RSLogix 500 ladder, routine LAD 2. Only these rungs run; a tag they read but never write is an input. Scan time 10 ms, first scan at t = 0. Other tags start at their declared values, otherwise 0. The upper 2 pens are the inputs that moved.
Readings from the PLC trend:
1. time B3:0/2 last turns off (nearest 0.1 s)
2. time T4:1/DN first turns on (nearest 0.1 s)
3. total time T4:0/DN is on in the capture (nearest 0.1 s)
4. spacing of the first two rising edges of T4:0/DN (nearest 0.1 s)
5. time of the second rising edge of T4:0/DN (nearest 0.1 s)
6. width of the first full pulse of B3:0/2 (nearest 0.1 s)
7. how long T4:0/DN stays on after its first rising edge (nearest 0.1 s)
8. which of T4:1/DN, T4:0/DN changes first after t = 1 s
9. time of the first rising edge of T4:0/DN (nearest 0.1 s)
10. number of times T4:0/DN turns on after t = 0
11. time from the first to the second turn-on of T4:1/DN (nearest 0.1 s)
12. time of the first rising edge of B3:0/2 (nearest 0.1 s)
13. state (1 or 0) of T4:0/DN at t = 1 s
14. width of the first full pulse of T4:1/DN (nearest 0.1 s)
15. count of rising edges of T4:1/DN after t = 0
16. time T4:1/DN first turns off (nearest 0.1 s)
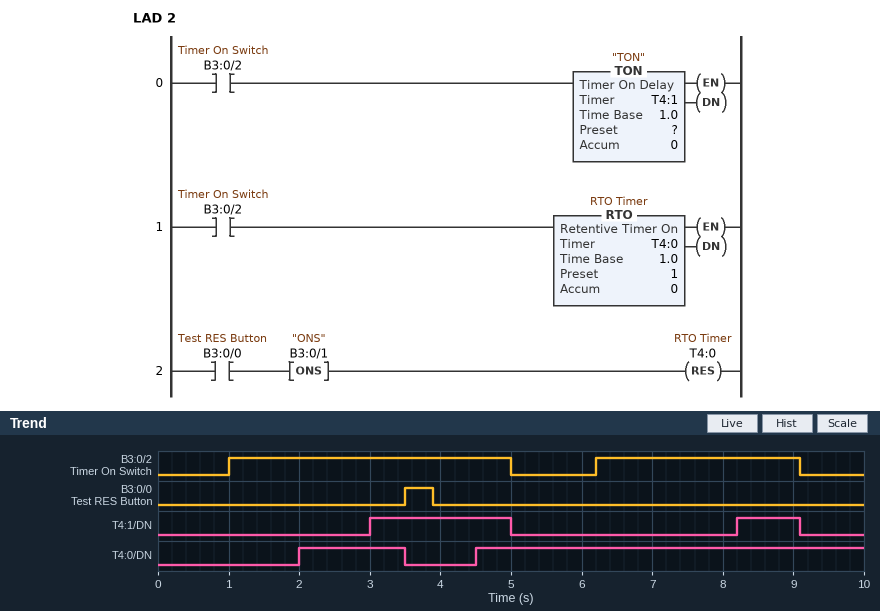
9.1 s
3.0 s
7.0 s
2.5 s
4.5 s
4.0 s
1.5 s
T4:0/DN
2.0 s
2
5.2 s
1.0 s
0
2.0 s
2
5.0 s
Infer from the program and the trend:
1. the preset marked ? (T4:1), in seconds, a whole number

2 s
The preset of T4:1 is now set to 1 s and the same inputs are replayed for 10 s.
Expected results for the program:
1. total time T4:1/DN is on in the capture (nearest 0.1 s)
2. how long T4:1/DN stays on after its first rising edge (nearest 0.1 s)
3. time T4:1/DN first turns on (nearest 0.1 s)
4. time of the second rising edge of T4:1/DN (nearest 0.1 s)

4.9 s
3.0 s
2.0 s
7.2 s
